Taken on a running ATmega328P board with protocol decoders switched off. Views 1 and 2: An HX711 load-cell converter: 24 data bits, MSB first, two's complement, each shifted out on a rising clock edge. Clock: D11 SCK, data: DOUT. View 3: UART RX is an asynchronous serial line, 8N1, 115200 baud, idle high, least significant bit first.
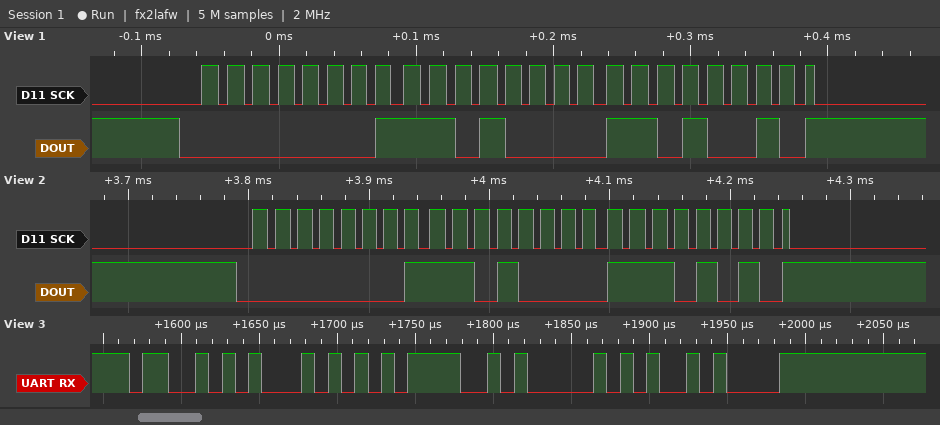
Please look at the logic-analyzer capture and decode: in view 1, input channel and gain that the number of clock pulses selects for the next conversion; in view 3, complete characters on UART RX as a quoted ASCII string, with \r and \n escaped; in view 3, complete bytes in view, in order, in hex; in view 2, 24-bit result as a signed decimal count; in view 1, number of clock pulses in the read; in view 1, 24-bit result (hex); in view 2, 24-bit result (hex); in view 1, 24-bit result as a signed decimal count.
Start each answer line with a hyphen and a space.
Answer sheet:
- channel A, gain 128
- "STOP\n"
- 53 54 4F 50 0A
- 119018
- 25
- 0x01D0D2
- 0x01D0EA
- 118994
